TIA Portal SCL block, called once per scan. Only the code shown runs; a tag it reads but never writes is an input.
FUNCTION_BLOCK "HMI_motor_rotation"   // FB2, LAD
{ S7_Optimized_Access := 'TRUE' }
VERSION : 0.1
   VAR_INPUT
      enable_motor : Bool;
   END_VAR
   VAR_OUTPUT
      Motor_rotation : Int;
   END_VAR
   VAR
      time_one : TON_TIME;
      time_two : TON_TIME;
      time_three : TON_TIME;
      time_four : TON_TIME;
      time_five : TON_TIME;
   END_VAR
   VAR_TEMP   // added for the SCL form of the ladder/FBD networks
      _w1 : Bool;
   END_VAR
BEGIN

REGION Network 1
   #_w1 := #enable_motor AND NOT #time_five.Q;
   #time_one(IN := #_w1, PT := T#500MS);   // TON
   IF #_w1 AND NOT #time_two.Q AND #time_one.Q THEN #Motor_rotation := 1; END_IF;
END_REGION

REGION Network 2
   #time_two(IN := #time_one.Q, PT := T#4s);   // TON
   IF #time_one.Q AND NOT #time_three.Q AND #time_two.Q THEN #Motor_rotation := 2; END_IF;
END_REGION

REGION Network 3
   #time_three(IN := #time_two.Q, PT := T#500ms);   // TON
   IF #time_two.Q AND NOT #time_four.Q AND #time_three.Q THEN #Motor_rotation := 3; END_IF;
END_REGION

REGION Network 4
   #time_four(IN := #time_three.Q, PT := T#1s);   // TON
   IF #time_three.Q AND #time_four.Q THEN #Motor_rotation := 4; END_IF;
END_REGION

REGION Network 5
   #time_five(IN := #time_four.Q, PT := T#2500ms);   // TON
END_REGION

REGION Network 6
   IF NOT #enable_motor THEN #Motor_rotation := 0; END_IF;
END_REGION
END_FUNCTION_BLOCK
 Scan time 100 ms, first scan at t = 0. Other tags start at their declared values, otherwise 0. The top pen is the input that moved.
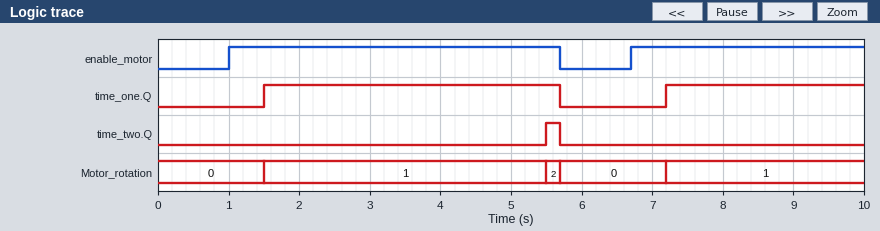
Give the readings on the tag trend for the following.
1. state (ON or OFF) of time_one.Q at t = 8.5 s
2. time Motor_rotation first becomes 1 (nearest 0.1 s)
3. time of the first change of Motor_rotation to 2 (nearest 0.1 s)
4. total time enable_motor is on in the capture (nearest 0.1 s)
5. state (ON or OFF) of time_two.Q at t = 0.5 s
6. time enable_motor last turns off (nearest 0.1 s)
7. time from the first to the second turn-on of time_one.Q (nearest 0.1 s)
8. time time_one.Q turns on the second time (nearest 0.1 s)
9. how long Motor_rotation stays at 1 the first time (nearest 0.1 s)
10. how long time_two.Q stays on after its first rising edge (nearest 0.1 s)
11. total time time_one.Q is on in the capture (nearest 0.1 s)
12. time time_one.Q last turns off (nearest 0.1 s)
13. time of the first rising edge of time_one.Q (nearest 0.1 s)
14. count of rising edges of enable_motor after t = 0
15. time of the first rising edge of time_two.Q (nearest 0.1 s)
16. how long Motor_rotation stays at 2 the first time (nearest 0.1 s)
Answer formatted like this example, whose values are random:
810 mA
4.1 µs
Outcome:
ON
1.5 s
5.5 s
8.0 s
OFF
5.7 s
5.7 s
7.2 s
4.0 s
0.2 s
7.0 s
5.7 s
1.5 s
2
5.5 s
0.2 s
